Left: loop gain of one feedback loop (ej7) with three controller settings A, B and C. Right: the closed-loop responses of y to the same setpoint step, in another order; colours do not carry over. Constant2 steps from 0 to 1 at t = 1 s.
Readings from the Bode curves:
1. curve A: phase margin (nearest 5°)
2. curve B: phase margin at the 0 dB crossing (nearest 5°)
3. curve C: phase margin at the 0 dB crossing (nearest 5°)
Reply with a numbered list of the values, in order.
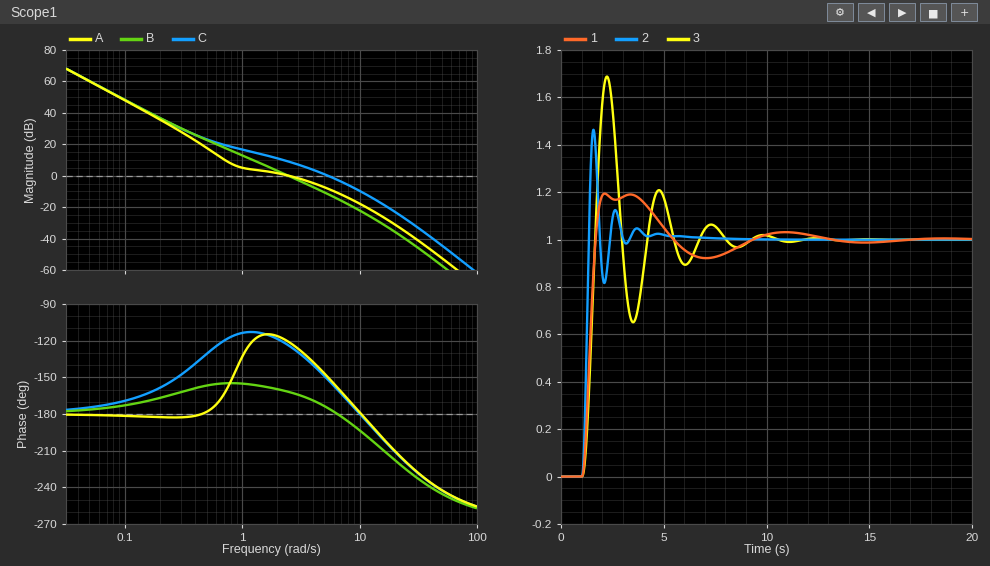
1. 60°
2. 20°
3. 30°
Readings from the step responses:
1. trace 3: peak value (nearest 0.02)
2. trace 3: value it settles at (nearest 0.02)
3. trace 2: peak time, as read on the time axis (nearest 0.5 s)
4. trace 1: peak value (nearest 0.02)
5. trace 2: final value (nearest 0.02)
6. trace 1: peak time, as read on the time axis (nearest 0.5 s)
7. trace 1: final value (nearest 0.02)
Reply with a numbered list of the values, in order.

1. 1.68
2. 1.00
3. 1.5 s
4. 1.20
5. 1.00
6. 2.0 s
7. 1.00
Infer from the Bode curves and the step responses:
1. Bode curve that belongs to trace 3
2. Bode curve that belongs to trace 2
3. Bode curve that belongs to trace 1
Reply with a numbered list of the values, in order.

1. B
2. C
3. A
